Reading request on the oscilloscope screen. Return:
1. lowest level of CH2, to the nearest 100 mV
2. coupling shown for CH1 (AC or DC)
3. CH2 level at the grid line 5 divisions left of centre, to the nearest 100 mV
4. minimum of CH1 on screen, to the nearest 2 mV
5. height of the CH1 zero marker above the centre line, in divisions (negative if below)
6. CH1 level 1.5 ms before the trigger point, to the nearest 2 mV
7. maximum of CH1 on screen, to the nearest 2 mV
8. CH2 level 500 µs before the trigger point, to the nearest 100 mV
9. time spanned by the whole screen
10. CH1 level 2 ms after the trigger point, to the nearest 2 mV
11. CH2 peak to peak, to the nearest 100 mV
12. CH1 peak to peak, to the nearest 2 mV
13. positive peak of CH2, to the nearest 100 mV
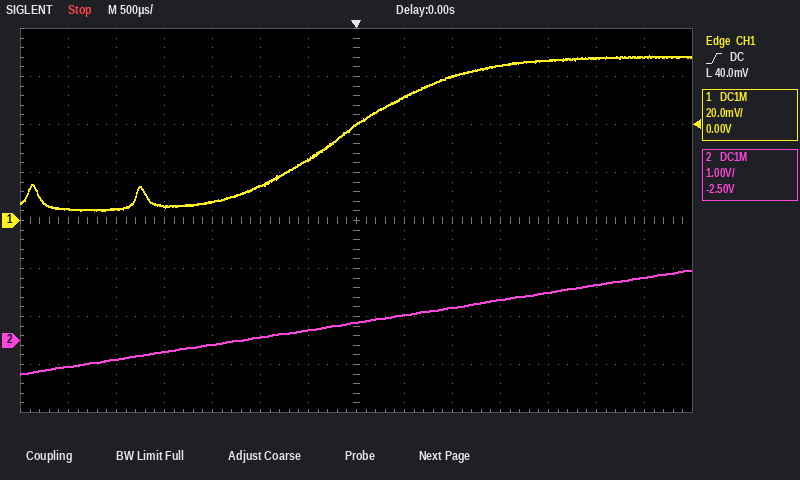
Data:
-700 mV
DC
-400 mV
4 mV
0.0 div
8 mV
68 mV
200 mV
7 ms
66 mV
2.2 V
64 mV
1.5 V
